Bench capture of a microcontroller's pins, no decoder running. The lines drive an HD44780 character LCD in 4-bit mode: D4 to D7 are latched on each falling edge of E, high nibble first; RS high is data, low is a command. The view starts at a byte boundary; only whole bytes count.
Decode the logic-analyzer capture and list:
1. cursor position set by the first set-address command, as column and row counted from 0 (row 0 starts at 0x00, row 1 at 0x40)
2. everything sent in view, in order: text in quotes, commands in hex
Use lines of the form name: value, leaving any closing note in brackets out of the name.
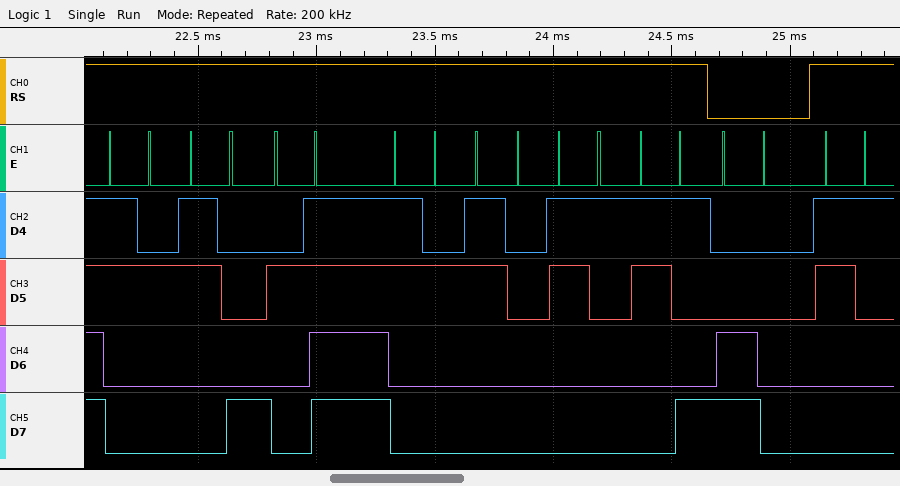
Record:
cursor position set by the first set-address command, as column and row counted from 0: column 0, row 1
everything sent in view, in order: text in quotes, commands in hex: "28/2019" 0xC0 "1"
